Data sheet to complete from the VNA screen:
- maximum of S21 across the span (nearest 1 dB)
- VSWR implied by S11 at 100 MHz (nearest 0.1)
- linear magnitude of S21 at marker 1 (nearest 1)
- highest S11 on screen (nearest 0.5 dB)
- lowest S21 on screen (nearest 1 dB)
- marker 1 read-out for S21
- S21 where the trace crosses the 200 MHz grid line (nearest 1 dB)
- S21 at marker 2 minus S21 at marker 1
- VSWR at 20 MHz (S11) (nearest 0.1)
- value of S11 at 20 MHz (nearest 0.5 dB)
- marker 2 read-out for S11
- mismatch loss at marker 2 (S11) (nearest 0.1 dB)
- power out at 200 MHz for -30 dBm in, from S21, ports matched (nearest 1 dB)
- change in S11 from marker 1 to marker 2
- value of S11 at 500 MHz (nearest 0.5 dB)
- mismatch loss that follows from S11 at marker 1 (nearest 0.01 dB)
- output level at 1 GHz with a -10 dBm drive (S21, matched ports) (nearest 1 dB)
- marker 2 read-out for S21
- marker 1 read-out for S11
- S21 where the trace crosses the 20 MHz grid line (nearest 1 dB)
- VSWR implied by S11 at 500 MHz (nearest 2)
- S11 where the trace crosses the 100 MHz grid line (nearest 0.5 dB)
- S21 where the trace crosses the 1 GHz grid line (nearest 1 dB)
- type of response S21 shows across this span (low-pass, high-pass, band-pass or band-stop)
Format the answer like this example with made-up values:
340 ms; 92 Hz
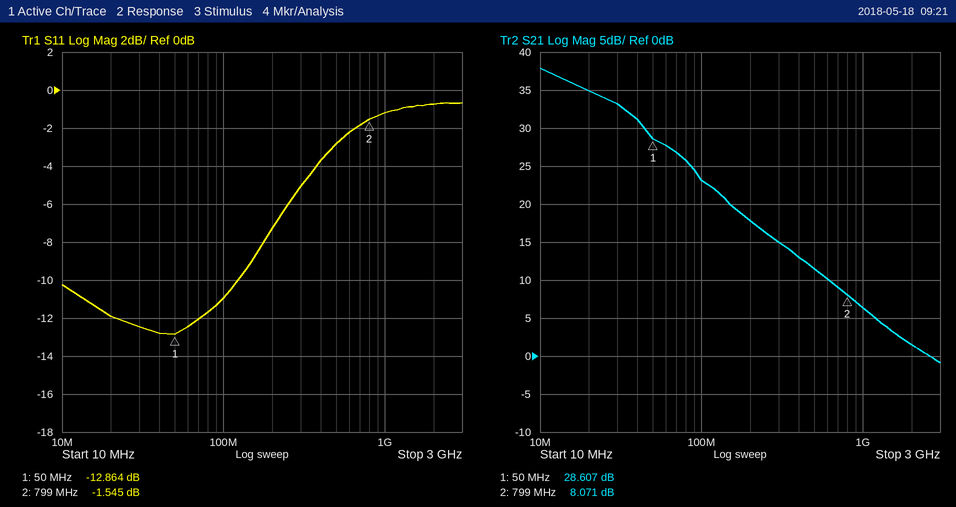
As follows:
38 dB; 1.8; 27; -0.5 dB; -1 dB; 28.607 dB; 18 dB; -20.536 dB; 1.7; -12.0 dB; -1.545 dB; 5.2 dB; -12 dBm; 11.319 dB; -3.0 dB; 0.23 dB; -4 dBm; 8.071 dB; -12.864 dB; 35 dB; 6; -11.0 dB; 6 dB; low-pass
